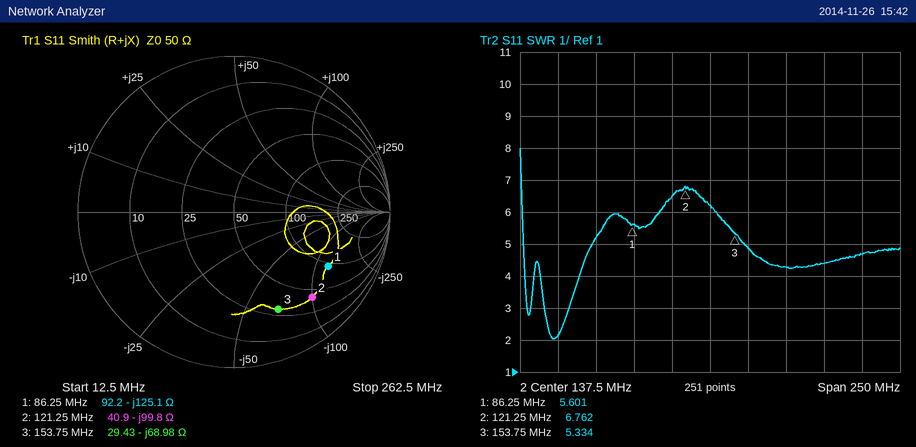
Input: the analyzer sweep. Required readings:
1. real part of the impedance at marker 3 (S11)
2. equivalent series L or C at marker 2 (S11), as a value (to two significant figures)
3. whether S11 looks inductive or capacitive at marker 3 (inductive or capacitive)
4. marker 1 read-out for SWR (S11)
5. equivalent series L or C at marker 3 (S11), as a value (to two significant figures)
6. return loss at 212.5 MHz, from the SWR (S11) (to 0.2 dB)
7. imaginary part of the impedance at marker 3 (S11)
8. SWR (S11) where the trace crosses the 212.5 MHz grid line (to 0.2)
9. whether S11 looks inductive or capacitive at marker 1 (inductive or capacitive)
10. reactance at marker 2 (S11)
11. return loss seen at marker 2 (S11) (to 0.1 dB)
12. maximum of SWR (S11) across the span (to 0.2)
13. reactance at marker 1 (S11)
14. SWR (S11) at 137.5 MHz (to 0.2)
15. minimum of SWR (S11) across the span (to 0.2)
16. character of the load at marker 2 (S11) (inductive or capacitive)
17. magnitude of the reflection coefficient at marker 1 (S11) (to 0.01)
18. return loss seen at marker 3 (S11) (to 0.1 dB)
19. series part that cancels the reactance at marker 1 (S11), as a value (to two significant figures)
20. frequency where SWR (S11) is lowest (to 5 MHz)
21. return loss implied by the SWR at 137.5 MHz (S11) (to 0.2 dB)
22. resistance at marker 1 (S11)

29.43 Ω
13 pF
capacitive
5.601
15 pF
4.0 dB
-68.98 Ω
4.4
capacitive
-99.8 Ω
2.6 dB
8.0
-125.1 Ω
6.2
2.0
capacitive
0.70
3.3 dB
230 nH
35 MHz
2.8 dB
92.2 Ω
